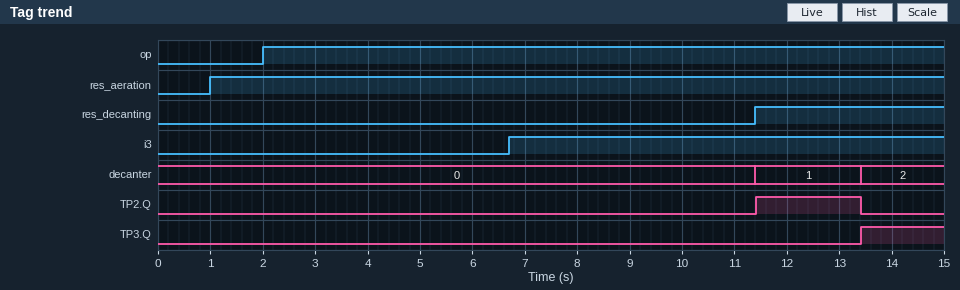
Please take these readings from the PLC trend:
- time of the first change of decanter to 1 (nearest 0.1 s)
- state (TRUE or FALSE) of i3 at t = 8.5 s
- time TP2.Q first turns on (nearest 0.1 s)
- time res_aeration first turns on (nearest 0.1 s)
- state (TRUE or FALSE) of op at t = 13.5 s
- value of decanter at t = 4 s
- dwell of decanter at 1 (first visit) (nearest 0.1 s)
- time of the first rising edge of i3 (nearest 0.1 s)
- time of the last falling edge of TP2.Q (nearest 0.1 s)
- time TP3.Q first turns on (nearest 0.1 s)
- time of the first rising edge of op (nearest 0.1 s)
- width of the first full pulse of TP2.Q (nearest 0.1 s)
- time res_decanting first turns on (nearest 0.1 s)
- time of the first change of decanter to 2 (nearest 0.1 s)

11.4 s
TRUE
11.4 s
1.0 s
TRUE
0
2.0 s
6.7 s
13.4 s
13.4 s
2.0 s
2.0 s
11.4 s
13.4 s
